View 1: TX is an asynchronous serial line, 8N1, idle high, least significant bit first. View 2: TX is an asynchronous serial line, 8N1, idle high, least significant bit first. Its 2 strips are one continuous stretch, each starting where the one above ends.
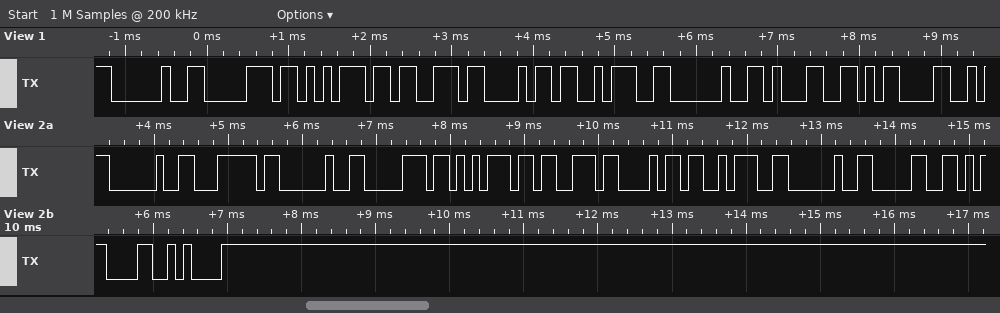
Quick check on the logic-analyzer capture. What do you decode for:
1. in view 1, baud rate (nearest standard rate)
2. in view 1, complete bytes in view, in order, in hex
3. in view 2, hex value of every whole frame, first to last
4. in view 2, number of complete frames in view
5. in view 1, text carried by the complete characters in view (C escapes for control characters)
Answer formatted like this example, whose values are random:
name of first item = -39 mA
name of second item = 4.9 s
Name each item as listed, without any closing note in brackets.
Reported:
in view 1, baud rate = 9600 baud
in view 1, complete bytes in view, in order, in hex = 0x20 0x70 0x75 0x73 0x68 0x3A 0x20 0x31 0x0D
in view 2, hex value of every whole frame, first to last = 20 7C 20 70 75 73 68 3A 20 30 0D 0A
in view 2, number of complete frames in view = 12
in view 1, text carried by the complete characters in view = " push: 1\r"
